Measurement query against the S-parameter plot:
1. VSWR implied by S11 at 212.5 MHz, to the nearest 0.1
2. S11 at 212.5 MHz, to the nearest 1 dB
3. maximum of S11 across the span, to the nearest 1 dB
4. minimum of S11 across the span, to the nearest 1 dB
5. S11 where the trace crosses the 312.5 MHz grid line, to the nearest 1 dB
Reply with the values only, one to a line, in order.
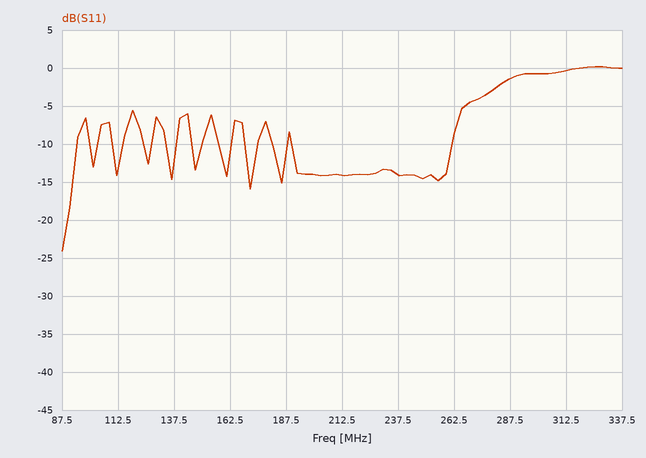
1.5
-14 dB
0 dB
-24 dB
0 dB
